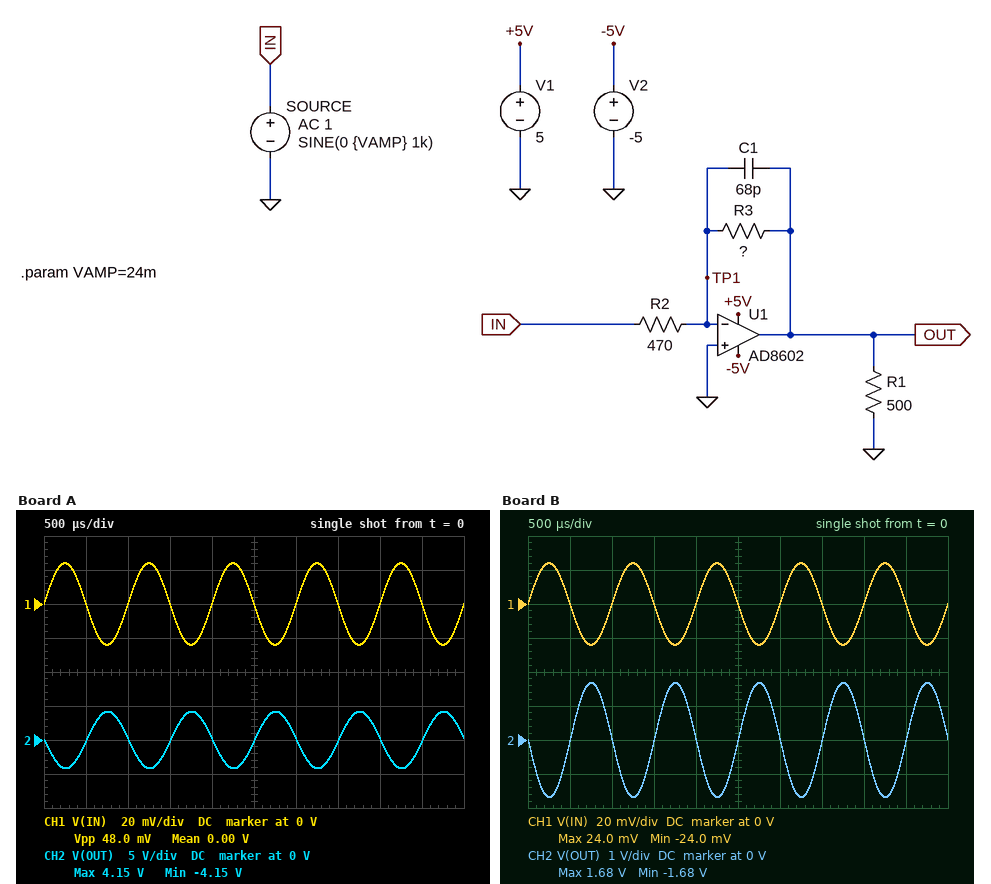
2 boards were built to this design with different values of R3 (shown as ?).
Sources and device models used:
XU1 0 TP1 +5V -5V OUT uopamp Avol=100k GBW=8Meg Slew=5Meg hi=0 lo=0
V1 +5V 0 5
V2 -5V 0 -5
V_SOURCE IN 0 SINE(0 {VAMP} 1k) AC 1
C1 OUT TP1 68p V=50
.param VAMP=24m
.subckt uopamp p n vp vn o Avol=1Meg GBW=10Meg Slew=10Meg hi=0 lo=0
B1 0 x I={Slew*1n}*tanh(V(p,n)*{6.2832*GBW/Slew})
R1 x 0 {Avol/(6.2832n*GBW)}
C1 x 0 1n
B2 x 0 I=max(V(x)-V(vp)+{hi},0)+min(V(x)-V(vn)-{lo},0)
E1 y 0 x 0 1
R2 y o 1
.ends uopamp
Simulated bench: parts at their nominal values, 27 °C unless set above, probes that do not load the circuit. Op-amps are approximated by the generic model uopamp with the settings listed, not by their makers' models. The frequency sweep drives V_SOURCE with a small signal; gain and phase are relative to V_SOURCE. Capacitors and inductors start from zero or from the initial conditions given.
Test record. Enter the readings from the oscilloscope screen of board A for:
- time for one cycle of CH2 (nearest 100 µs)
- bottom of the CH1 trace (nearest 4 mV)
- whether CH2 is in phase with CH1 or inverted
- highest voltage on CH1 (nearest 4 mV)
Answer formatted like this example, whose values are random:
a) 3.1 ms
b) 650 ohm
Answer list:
a) 1.0 ms
b) -24 mV
c) inverted
d) 24 mV
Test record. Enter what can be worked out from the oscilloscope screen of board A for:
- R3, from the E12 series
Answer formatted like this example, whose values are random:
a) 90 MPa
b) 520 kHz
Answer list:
a) 82 kΩ
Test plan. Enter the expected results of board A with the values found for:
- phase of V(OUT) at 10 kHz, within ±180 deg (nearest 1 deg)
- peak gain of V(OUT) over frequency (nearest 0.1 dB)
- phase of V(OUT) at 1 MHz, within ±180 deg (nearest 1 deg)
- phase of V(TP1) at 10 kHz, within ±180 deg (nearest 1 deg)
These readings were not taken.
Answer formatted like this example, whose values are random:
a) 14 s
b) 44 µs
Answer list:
a) 150 deg
b) 44.8 dB
c) 87 deg
d) 60 deg
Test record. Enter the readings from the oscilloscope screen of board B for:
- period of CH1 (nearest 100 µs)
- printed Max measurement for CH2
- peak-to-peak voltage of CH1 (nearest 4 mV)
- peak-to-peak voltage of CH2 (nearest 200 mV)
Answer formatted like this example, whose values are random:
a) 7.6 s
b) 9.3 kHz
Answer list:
a) 1.0 ms
b) 1.68 V
c) 48 mV
d) 3.4 V
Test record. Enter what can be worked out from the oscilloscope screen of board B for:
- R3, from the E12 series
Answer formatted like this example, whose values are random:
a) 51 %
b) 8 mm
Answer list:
a) 33 kΩ
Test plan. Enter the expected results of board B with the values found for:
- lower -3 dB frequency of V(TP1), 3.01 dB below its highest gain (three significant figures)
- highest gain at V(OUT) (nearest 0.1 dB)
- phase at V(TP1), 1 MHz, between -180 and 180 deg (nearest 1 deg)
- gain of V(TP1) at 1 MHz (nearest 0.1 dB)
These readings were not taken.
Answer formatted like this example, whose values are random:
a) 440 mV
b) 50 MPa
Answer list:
a) 43.3 kHz
b) 36.9 dB
c) -2 deg
d) -8.4 dB
